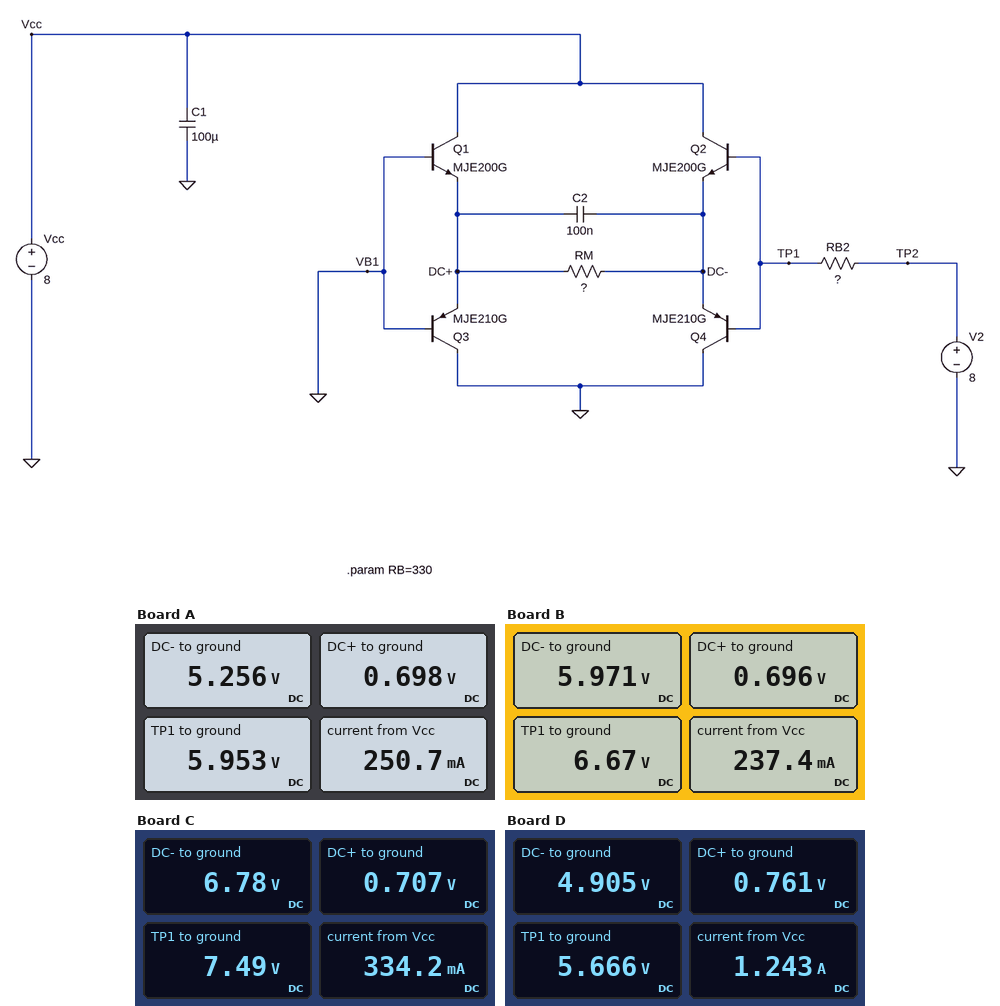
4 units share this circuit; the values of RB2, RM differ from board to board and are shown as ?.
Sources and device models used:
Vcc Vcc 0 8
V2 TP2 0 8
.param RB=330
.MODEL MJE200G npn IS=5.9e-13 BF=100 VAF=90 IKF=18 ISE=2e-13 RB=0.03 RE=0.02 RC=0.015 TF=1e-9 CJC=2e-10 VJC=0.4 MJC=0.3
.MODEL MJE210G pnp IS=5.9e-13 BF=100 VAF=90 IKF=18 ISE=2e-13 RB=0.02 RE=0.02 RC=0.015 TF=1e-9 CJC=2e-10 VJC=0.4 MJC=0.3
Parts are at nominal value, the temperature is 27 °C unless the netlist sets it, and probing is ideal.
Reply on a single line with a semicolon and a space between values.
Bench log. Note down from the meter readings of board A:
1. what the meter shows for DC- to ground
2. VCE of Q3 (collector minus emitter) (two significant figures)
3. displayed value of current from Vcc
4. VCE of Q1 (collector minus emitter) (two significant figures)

5.256 V; -700 mV; 250.7 mA; 7.3 V
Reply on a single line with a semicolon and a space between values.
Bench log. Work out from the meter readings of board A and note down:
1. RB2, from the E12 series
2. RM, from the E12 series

820 Ω; 18 Ω
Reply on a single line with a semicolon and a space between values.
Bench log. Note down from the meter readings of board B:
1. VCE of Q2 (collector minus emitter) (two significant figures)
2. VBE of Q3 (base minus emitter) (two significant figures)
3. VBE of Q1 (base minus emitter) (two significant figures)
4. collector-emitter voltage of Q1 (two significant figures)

2.0 V; -700 mV; -700 mV; 7.3 V
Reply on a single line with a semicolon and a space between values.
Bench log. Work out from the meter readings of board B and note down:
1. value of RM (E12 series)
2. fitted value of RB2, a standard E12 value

22 Ω; 560 Ω
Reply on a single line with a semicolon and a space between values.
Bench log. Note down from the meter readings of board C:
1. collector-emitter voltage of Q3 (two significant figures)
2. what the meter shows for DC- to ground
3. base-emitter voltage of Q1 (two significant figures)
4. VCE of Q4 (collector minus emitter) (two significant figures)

-710 mV; 6.78 V; -710 mV; -6.8 V
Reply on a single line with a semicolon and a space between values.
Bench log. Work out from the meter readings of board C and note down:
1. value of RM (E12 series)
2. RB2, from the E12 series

18 Ω; 150 Ω
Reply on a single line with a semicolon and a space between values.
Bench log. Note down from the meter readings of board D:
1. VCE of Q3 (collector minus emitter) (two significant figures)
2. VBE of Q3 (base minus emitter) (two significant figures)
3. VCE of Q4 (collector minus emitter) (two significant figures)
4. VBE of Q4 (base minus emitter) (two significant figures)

-760 mV; -760 mV; -4.9 V; 760 mV
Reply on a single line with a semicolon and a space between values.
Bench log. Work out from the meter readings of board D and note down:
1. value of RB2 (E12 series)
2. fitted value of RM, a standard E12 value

180 Ω; 3.3 Ω
